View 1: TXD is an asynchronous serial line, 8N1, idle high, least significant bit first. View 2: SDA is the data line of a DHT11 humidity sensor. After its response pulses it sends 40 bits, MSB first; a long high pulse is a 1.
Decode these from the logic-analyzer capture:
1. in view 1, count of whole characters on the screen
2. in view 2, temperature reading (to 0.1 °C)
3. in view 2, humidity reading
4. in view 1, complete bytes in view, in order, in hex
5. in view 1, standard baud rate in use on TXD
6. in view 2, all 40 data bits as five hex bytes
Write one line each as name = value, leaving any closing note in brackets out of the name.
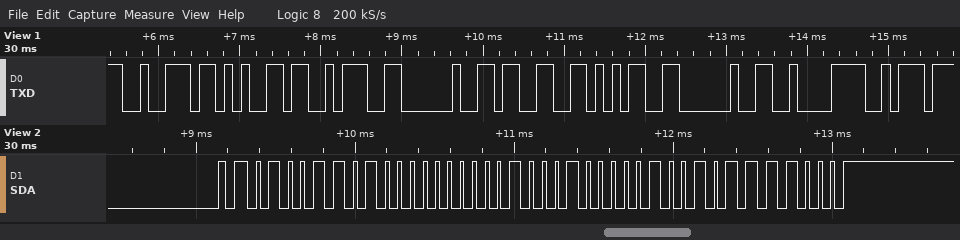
in view 1, count of whole characters on the screen = 9
in view 2, temperature reading = 34.9 °C
in view 2, humidity reading = 77 %
in view 1, complete bytes in view, in order, in hex = 72 65 3A 20 33 35 20 C2 BA
in view 1, standard baud rate in use on TXD = 9600 baud
in view 2, all 40 data bits as five hex bytes = 4D 00 22 09 78
